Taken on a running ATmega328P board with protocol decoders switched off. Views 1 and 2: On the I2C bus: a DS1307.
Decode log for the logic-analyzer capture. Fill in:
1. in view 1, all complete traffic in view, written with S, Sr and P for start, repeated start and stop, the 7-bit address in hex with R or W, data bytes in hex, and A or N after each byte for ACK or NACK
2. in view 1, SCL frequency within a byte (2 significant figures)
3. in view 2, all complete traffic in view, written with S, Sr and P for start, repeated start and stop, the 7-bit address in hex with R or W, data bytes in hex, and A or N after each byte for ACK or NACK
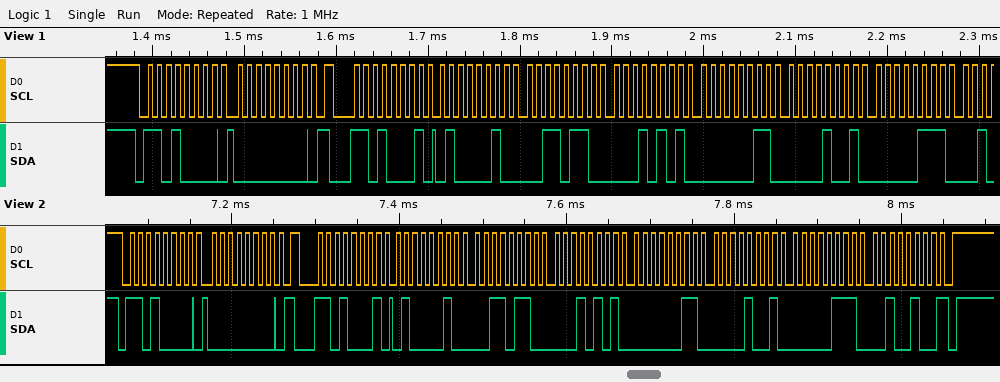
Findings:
S 68W A 00 A Sr 68R A 42 A 36 A 15 A 03 A 09 A 07 A
100 kHz
S 68W A 00 A Sr 68R A 42 A 36 A 15 A 03 A 09 A 07 A 24 N P
